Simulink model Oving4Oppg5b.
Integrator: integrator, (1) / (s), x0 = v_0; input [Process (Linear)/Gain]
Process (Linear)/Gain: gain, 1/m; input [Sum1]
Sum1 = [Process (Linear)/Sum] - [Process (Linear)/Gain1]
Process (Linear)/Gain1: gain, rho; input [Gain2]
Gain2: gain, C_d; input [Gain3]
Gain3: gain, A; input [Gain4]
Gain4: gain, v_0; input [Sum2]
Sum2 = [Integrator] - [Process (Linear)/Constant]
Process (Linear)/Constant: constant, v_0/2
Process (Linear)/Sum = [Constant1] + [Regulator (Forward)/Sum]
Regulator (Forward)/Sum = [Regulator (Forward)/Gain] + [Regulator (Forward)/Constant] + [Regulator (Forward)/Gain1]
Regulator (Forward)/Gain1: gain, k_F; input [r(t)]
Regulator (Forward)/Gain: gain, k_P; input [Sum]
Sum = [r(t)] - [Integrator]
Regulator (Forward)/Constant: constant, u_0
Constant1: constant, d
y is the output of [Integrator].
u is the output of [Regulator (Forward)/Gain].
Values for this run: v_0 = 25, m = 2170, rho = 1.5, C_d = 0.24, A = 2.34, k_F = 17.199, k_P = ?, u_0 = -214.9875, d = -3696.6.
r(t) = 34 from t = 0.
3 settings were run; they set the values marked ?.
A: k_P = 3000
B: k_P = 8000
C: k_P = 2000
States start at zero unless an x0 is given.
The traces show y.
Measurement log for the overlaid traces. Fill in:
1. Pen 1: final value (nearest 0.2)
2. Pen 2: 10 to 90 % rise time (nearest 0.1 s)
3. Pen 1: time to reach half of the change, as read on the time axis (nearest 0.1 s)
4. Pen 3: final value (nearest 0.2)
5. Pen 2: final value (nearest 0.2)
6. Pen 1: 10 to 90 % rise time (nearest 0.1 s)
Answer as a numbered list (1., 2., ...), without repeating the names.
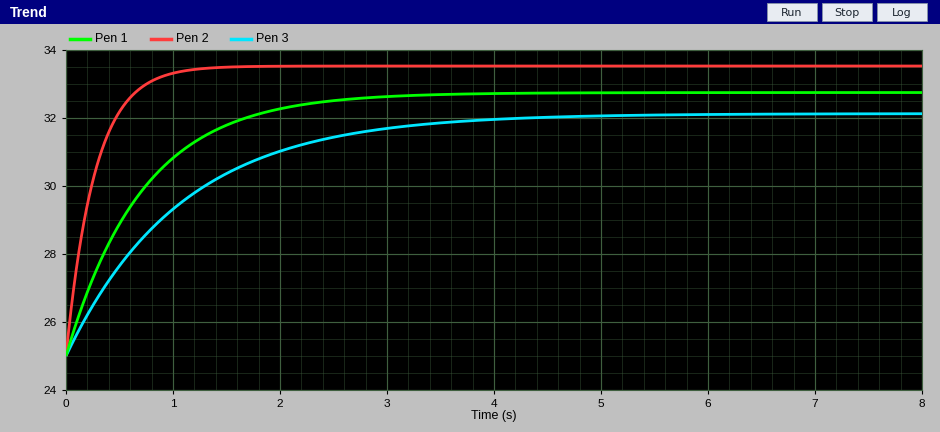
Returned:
1. 32.8
2. 0.6 s
3. 0.5 s
4. 32.2
5. 33.6
6. 1.6 s
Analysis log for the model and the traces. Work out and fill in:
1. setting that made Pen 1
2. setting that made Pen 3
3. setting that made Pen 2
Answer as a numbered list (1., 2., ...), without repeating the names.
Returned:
1. A
2. C
3. B
